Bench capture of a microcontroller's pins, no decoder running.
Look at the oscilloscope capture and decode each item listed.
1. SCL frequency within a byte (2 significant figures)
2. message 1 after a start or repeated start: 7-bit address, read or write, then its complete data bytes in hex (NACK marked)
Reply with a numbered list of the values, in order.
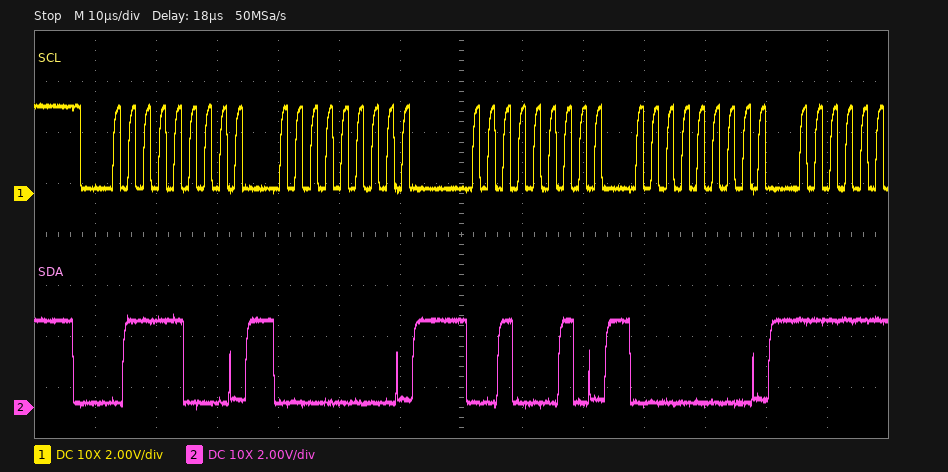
1. 400 kHz
2. 0x3C write: 00 22 00
